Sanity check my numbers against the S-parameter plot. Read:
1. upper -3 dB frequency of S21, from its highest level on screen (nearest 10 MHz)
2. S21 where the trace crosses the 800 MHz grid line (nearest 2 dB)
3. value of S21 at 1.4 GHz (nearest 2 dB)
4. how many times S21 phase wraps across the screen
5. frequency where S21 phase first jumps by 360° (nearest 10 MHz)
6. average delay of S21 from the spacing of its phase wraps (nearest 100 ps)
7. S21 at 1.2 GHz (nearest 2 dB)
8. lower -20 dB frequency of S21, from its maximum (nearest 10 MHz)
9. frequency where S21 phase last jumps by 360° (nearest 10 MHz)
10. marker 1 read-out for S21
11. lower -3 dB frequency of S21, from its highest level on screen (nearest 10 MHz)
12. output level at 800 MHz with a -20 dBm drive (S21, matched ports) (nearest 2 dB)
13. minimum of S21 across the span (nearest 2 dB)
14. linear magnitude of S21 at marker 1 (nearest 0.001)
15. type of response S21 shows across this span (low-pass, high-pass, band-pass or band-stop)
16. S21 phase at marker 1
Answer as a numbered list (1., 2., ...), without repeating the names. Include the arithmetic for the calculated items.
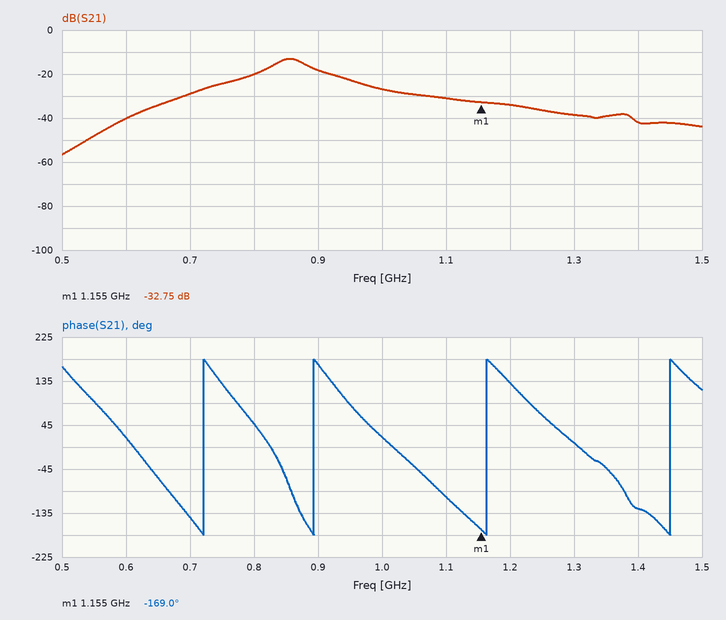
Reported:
1. 880 MHz
2. -20 dB
3. -42 dB
4. 4
5. 720 MHz
6. 3 cycles / (1.45 GHz − 720 MHz) ≈ 4.1 ns
7. -34 dB
8. 660 MHz
9. 1.45 GHz
10. -32.75 dB
11. 830 MHz
12. -20 dBm + (-20 dB) = -40 dBm
13. -56 dB
14. 10^(-32.75/20) ≈ 0.023
15. band-pass
16. -169.0°
